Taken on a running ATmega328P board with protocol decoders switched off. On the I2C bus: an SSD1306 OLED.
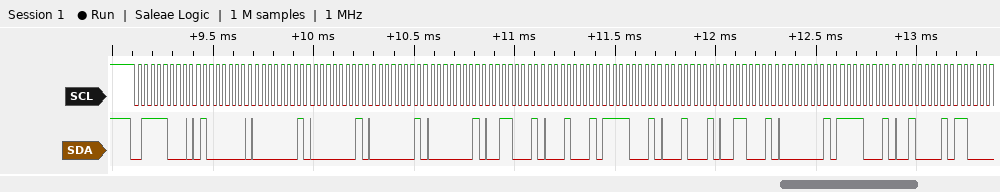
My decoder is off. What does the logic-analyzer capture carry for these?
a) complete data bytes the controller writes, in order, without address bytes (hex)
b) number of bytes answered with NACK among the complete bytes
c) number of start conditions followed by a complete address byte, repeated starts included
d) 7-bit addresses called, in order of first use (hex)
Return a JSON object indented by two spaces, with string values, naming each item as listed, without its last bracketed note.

{
  "complete data bytes the controller writes, in order, without address bytes": "40 01 01 01 01 31 11 F1 11 31 01 F1 21",
  "number of bytes answered with NACK among the complete bytes": "0",
  "number of start conditions followed by a complete address byte, repeated starts included": "1",
  "7-bit addresses called, in order of first use": "0x3C"
}
